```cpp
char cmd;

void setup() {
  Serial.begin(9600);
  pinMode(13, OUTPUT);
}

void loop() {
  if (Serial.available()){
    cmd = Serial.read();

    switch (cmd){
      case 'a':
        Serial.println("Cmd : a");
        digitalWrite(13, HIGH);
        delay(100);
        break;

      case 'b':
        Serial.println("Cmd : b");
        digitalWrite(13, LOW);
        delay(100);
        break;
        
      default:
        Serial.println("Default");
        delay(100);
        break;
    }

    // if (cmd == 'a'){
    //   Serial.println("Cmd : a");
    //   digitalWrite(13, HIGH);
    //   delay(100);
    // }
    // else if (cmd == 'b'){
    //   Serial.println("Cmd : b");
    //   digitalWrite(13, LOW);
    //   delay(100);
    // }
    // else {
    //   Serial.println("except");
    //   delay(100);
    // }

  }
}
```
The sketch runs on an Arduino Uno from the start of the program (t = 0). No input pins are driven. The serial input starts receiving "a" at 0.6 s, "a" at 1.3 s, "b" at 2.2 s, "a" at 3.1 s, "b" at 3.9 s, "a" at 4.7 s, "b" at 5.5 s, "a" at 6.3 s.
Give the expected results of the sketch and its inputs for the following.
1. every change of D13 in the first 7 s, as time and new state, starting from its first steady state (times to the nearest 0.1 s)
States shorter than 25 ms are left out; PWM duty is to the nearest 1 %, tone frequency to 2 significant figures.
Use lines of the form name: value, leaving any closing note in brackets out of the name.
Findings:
every change of D13 in the first 7 s, as time and new state, starting from its first steady state: 0 s low; 0.6 s high; 2.2 s low; 3.1 s high; 3.9 s low; 4.7 s high; 5.5 s low; 6.3 s high
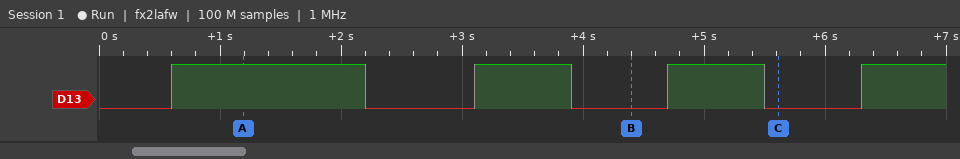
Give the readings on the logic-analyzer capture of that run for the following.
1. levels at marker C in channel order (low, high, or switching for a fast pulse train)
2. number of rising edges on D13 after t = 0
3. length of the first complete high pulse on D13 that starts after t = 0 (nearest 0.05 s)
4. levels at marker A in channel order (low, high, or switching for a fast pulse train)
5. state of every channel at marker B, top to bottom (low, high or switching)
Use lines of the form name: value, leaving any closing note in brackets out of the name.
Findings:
levels at marker C in channel order: D13 low
number of rising edges on D13 after t = 0: 4
length of the first complete high pulse on D13 that starts after t = 0: 1.60 s
levels at marker A in channel order: D13 high
state of every channel at marker B, top to bottom: D13 low
